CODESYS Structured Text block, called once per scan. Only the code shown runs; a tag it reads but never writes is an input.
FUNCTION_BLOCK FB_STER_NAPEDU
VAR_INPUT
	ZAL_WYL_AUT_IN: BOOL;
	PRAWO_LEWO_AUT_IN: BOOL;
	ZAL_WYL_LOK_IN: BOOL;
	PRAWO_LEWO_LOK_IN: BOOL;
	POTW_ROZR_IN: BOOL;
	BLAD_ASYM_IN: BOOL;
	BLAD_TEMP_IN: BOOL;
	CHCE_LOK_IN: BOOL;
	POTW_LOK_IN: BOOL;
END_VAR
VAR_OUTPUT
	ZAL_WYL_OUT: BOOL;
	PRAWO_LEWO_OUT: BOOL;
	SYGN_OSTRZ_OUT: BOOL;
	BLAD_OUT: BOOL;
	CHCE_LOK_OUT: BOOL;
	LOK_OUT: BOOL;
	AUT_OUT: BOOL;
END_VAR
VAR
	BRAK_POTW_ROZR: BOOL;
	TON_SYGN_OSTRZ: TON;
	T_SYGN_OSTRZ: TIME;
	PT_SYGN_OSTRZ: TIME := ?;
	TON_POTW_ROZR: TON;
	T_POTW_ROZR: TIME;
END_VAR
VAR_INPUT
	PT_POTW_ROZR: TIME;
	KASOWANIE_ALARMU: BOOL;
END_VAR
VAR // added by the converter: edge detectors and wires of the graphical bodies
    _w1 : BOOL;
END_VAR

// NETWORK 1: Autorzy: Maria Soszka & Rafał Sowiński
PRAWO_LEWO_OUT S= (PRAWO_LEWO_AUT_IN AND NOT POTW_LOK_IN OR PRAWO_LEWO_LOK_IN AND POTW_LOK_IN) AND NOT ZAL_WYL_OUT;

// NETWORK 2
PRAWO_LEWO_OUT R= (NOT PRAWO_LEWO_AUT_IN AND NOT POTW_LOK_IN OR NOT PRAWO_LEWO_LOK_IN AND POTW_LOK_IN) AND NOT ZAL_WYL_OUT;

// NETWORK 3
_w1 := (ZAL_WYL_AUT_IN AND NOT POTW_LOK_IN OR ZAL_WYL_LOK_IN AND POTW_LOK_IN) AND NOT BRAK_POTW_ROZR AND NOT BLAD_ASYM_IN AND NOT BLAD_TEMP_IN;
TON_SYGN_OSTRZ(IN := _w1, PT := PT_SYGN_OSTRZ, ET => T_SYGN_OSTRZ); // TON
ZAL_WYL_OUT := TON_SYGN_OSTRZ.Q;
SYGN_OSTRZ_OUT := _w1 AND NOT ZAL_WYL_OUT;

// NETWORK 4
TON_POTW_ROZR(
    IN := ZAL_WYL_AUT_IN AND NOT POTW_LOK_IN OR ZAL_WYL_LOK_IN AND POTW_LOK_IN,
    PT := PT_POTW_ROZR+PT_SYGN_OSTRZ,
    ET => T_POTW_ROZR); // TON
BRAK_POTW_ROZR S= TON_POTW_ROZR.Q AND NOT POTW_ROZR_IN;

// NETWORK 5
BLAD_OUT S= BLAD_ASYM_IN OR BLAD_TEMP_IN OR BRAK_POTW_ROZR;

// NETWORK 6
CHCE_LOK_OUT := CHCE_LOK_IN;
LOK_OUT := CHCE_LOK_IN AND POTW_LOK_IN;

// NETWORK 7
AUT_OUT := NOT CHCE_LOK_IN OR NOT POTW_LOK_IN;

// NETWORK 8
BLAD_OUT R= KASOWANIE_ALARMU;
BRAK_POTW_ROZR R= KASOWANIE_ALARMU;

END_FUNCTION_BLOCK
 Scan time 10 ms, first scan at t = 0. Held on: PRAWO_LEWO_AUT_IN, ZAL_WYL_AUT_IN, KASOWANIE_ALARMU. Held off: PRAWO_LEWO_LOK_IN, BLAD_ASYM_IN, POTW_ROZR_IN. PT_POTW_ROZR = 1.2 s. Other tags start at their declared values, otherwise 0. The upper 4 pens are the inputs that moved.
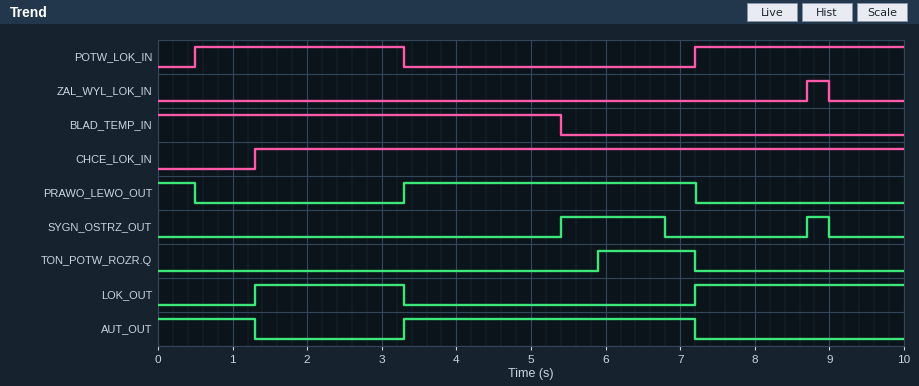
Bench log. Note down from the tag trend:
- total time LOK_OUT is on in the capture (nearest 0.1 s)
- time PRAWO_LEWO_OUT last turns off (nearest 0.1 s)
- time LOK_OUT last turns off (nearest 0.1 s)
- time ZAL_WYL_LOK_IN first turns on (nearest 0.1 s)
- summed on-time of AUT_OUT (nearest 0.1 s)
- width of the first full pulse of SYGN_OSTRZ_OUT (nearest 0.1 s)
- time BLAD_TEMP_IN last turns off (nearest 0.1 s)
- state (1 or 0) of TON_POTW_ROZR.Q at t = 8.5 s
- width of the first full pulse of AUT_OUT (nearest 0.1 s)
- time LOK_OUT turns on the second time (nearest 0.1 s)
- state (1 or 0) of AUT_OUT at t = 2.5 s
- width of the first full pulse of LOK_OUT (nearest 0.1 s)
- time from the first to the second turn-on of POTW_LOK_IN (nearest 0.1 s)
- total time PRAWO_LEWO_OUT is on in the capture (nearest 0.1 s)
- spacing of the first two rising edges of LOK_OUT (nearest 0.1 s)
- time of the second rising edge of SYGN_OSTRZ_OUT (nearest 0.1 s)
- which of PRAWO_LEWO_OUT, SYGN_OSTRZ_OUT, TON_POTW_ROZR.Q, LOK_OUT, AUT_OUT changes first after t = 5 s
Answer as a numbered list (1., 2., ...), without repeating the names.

1. 4.8 s
2. 7.2 s
3. 3.3 s
4. 8.7 s
5. 5.2 s
6. 1.4 s
7. 5.4 s
8. 0
9. 3.9 s
10. 7.2 s
11. 0
12. 2.0 s
13. 6.7 s
14. 4.4 s
15. 5.9 s
16. 8.7 s
17. SYGN_OSTRZ_OUT
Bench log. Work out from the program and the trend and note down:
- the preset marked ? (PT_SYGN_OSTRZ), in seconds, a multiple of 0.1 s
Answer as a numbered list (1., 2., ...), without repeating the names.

1. 1.4 s
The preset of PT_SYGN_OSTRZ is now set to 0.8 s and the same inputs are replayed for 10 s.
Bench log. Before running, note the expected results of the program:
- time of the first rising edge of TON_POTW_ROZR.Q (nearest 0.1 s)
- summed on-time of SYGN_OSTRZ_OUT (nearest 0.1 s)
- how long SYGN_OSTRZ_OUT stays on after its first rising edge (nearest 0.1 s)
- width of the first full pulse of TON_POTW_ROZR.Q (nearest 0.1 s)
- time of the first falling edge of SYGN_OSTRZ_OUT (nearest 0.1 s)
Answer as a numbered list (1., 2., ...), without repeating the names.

1. 5.3 s
2. 1.1 s
3. 0.8 s
4. 1.9 s
5. 6.2 s
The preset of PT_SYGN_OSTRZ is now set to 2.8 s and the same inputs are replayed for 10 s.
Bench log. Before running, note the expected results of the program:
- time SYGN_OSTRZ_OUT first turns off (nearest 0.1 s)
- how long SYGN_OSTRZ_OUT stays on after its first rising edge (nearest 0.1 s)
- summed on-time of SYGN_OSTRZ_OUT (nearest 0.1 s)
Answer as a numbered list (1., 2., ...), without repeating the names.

1. 7.2 s
2. 1.8 s
3. 2.1 s
